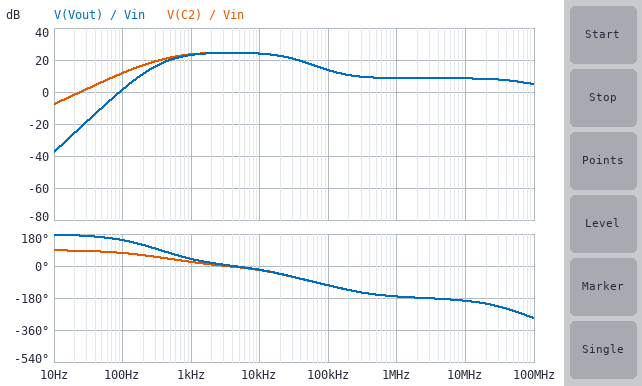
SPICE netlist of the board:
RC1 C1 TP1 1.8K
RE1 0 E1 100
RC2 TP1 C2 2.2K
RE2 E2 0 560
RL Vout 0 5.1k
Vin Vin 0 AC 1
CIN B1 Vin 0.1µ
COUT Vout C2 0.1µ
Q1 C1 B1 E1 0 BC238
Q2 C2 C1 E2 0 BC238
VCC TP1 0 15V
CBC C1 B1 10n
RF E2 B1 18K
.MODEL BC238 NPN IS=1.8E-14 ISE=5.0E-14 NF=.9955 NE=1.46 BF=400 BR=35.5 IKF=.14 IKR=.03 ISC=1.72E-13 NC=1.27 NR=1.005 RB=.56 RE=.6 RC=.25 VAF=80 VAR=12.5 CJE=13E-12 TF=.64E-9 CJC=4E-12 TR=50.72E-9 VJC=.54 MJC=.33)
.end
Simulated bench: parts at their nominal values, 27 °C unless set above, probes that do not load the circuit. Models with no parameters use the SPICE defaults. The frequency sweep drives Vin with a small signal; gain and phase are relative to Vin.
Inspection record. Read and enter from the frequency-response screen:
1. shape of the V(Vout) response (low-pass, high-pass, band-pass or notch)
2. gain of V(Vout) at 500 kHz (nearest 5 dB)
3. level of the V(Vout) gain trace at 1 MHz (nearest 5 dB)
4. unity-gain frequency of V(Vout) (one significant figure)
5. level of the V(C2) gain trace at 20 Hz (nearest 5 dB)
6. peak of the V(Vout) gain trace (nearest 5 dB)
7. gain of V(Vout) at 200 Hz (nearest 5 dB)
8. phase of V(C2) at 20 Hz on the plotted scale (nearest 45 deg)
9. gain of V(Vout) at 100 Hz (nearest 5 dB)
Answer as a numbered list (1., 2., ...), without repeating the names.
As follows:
1. band-pass
2. 10 dB
3. 10 dB
4. 90 Hz
5. 0 dB
6. 25 dB
7. 10 dB
8. 90 deg
9. 0 dB
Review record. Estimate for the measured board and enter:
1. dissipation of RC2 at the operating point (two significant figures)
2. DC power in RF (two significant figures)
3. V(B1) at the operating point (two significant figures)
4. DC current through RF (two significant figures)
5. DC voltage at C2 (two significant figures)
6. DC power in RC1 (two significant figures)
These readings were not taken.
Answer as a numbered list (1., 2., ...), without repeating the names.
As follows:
1. 23 mW
2. 9.8 µW
3. 1.4 V
4. 23 µA
5. 7.9 V
6. 87 mW
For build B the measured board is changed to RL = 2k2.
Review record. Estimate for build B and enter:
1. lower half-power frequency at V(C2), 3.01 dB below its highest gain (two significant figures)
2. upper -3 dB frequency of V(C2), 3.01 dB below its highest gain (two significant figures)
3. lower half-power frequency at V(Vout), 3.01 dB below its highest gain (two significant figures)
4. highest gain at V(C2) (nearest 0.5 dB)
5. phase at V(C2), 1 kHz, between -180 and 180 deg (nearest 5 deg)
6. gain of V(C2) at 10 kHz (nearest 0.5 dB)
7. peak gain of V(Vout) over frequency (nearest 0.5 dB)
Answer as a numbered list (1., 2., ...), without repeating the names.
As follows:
1. 270 Hz
2. 25 kHz
3. 720 Hz
4. 22.0 dB
5. 10 deg
6. 21.0 dB
7. 21.5 dB
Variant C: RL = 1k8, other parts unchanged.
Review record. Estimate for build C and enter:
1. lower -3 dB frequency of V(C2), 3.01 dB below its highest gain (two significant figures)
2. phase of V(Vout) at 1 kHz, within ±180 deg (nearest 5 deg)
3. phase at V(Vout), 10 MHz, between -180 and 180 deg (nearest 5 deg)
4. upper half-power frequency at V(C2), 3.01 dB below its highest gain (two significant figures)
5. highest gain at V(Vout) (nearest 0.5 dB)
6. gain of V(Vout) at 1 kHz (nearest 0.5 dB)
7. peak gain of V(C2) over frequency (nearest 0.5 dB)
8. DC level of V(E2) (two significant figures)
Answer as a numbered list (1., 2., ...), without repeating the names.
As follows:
1. 250 Hz
2. 50 deg
3. 170 deg
4. 22 kHz
5. 20.5 dB
6. 19.0 dB
7. 21.5 dB
8. 1.8 V
